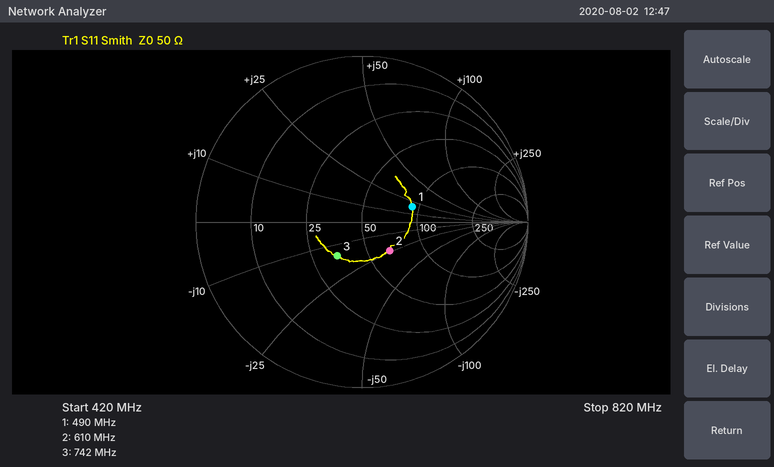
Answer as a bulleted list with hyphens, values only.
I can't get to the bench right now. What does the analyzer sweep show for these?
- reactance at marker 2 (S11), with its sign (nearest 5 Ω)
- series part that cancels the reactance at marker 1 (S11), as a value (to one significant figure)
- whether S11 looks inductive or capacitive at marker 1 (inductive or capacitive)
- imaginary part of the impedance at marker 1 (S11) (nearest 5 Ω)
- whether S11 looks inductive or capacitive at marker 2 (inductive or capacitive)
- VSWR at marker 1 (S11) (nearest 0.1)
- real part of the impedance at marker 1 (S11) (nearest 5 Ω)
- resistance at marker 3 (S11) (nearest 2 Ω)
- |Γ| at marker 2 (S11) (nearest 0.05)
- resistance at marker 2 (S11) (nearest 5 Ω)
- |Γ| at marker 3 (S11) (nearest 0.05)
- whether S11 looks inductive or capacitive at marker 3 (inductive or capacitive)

- -25 Ω
- 20 pF
- inductive
- +20 Ω
- capacitive
- 1.9
- 90 Ω
- 34 Ω
- 0.25
- 65 Ω
- 0.25
- capacitive
